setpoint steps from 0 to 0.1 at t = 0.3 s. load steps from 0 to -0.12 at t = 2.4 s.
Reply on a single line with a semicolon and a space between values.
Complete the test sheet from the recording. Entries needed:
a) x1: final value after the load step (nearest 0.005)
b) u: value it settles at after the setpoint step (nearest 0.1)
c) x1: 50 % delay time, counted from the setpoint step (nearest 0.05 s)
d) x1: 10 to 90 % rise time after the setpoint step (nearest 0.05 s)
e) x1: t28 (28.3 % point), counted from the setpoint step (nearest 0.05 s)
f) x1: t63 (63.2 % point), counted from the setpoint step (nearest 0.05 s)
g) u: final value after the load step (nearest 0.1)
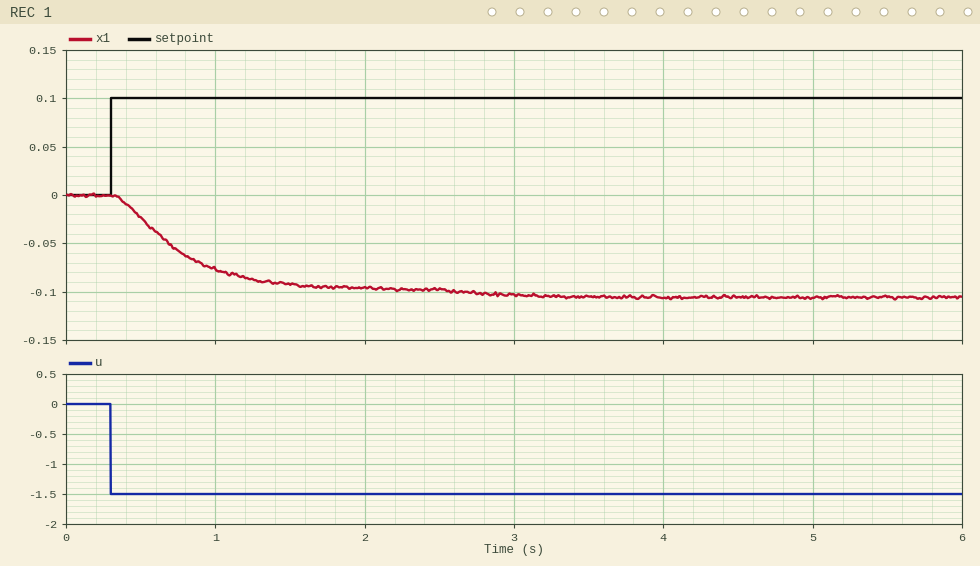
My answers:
-0.105; -1.5; 0.40 s; 0.85 s; 0.25 s; 0.50 s; -1.5
